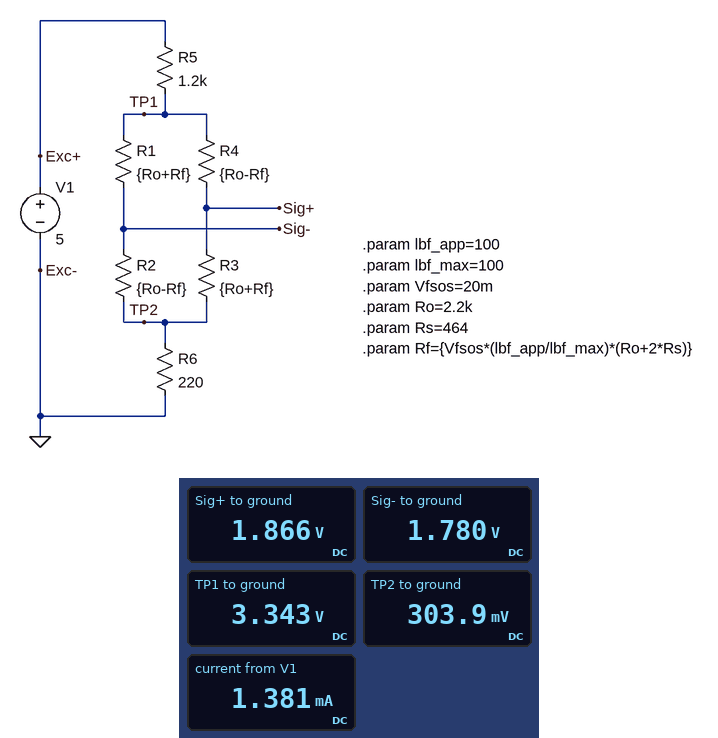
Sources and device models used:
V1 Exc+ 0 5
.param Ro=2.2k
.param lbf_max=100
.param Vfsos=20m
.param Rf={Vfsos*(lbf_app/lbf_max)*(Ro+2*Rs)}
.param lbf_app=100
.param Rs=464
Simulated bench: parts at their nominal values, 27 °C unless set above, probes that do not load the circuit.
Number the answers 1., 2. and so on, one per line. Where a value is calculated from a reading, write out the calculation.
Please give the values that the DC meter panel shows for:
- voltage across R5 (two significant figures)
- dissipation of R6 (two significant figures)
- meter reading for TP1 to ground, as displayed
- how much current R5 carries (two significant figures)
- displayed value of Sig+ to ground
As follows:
1. 5 V - 3.343 V = 1.7 V
2. (303.9 mV)^2 / 220 Ω = 420 µW
3. 3.343 V
4. (5 V - 3.343 V) / 1.2 kΩ = 1.4 mA
5. 1.866 V
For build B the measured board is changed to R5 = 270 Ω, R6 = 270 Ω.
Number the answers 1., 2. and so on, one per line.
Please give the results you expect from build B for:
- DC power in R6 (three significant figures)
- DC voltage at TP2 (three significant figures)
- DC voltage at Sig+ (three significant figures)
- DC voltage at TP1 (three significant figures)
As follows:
1. 899 µW
2. 493 mV
3. 2.56 V
4. 4.51 V
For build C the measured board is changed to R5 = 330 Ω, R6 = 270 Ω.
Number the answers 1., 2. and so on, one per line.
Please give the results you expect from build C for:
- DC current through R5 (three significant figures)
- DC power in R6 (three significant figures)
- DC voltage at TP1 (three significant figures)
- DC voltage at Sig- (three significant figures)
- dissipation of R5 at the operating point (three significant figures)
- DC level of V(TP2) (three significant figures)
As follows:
1. 1.79 mA
2. 861 µW
3. 4.41 V
4. 2.39 V
5. 1.05 mW
6. 482 mV
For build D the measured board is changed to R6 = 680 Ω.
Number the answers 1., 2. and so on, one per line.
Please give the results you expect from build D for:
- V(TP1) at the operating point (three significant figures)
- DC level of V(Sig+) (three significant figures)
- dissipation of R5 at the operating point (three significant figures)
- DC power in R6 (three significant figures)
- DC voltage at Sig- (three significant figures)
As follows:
1. 3.53 V
2. 2.22 V
3. 1.80 mW
4. 1.02 mW
5. 2.14 V
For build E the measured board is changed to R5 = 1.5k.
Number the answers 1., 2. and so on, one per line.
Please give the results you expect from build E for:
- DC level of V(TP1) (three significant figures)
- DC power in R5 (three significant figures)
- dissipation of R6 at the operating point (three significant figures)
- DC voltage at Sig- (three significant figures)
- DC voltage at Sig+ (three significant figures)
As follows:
1. 3.09 V
2. 2.44 mW
3. 358 µW
4. 1.64 V
5. 1.72 V
